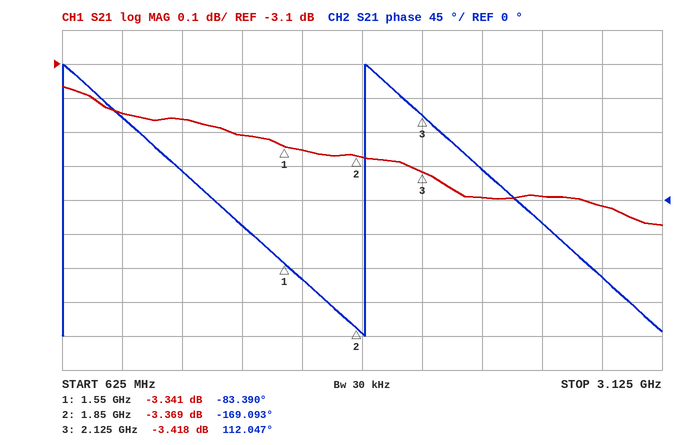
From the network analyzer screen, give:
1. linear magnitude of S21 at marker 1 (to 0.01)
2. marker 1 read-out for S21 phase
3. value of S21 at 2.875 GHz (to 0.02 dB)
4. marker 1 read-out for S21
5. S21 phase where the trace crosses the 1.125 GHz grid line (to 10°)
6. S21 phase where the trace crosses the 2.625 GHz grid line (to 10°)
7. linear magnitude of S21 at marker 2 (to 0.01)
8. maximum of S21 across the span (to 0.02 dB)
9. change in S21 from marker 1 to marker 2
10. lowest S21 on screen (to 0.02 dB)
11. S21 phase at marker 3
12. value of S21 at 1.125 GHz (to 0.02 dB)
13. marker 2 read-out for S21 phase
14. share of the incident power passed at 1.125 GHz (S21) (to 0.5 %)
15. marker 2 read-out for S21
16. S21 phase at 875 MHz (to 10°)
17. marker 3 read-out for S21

0.68
-83.390°
-3.52 dB
-3.341 dB
40°
-30°
0.68
-3.16 dB
-0.028 dB
-3.58 dB
112.047°
-3.26 dB
-169.093°
47.0 %
-3.369 dB
110°
-3.418 dB
